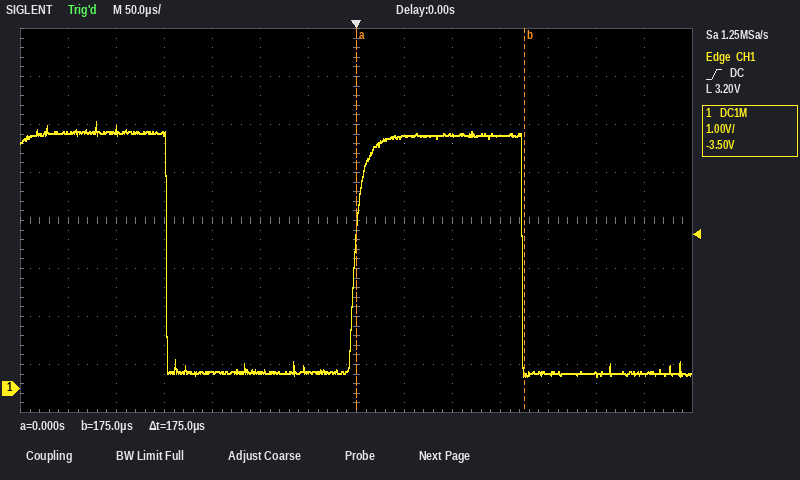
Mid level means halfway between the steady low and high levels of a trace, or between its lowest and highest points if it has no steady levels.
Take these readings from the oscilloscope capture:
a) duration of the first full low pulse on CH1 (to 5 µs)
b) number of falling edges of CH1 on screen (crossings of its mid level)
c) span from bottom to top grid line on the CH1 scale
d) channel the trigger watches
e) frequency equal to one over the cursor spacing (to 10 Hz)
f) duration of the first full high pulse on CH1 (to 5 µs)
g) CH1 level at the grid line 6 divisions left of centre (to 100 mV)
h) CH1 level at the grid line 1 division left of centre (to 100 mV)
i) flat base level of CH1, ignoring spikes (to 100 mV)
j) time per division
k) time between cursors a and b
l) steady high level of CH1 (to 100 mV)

195 µs
2
8 V
CH1
5.71 kHz
175 µs
5.3 V
300 mV
300 mV
50 µs
175 µs
5.3 V
